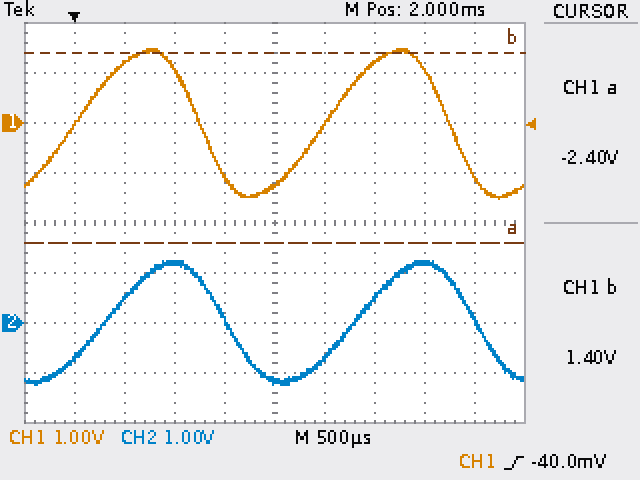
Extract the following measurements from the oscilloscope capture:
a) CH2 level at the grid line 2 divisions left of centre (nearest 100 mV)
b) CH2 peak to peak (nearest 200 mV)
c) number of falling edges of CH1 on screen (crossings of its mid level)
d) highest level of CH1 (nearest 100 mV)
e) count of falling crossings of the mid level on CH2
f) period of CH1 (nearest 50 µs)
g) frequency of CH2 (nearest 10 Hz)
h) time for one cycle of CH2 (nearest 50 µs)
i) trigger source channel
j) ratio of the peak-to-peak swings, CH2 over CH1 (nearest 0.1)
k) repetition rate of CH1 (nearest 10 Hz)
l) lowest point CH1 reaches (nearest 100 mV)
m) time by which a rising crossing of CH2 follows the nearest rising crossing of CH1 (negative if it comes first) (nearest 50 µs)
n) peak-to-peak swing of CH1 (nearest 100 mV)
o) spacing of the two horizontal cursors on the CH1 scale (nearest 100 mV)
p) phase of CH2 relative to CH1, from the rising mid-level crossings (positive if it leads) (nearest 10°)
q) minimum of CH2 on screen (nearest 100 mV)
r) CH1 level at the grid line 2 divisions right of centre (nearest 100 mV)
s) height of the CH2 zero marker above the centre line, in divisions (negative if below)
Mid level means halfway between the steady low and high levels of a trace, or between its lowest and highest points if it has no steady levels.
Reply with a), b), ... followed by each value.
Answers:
a) 1.2 V
b) 2.4 V
c) 2
d) 1.5 V
e) 2
f) 2.50 ms
g) 400 Hz
h) 2.50 ms
i) CH1
j) 0.8
k) 400 Hz
l) -1.5 V
m) +300 µs
n) 3.0 V
o) 3.8 V
p) -40°
q) -1.2 V
r) 1.2 V
s) -2.0 div
